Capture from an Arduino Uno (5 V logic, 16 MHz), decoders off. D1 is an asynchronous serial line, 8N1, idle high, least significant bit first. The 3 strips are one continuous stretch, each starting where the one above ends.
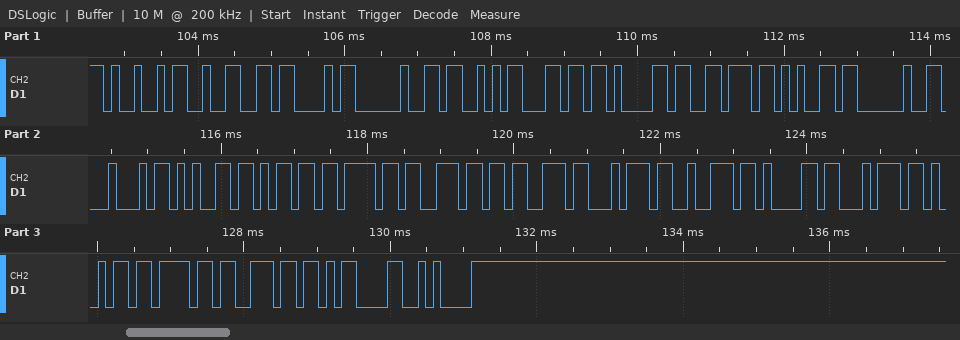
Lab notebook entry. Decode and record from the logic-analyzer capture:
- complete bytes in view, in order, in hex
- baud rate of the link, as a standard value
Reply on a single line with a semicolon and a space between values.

0x49 0x32 0x43 0x20 0x53 0x6C 0x61 0x76 0x65 0x20 0x44 0x65 0x6D 0x6F 0x6E 0x73 0x74 0x72 0x61 0x74 0x69 0x6F 0x6E 0x0D 0x0A; 9600 baud
